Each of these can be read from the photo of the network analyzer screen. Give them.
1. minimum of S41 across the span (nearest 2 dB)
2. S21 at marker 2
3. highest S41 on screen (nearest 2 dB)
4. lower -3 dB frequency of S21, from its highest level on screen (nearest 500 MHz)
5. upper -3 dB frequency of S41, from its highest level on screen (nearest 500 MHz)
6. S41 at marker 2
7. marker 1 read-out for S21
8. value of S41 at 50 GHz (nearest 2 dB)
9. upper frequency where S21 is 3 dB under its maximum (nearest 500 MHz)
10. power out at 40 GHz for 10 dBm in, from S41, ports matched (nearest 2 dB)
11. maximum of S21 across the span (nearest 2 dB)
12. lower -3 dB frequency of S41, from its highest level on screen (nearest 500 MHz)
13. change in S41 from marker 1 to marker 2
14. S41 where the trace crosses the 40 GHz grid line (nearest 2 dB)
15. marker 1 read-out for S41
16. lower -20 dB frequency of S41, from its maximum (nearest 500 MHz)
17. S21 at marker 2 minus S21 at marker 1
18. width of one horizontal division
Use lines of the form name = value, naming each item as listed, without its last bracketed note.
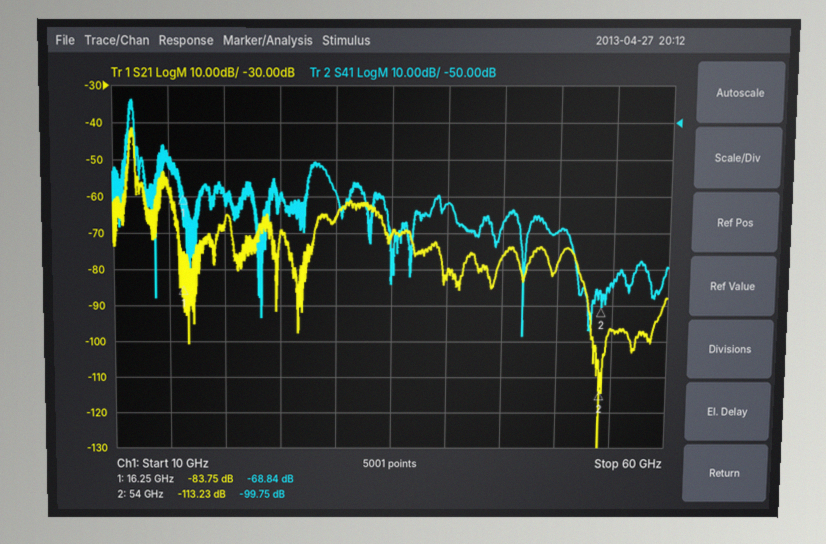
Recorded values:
minimum of S41 across the span = -108 dB
S21 at marker 2 = -113.23 dB
highest S41 on screen = -44 dB
lower -3 dB frequency of S21, from its highest level on screen = 11.5 GHz
upper -3 dB frequency of S41, from its highest level on screen = 12.0 GHz
S41 at marker 2 = -99.75 dB
marker 1 read-out for S21 = -83.75 dB
value of S41 at 50 GHz = -80 dB
upper frequency where S21 is 3 dB under its maximum = 12.0 GHz
power out at 40 GHz for 10 dBm in, from S41, ports matched = -62 dBm
maximum of S21 across the span = -42 dB
lower -3 dB frequency of S41, from its highest level on screen = 11.5 GHz
change in S41 from marker 1 to marker 2 = -30.91 dB
S41 where the trace crosses the 40 GHz grid line = -72 dB
marker 1 read-out for S41 = -68.84 dB
lower -20 dB frequency of S41, from its maximum = 11.0 GHz
S21 at marker 2 minus S21 at marker 1 = -29.48 dB
width of one horizontal division = 5 GHz
